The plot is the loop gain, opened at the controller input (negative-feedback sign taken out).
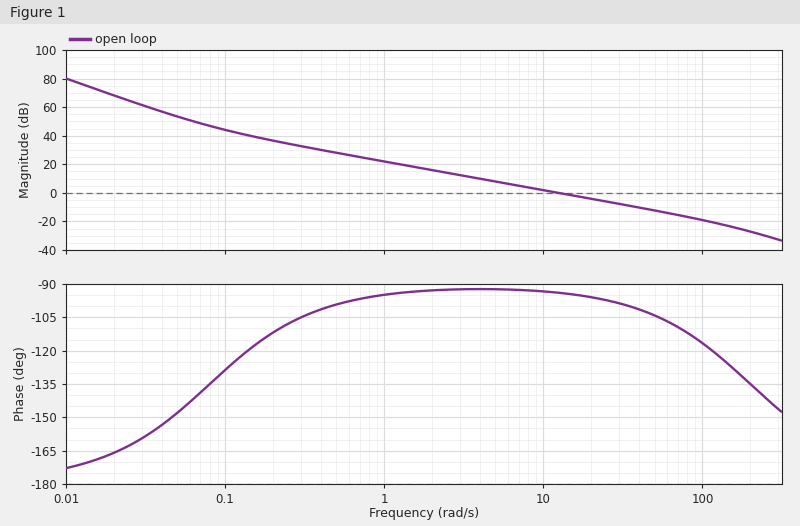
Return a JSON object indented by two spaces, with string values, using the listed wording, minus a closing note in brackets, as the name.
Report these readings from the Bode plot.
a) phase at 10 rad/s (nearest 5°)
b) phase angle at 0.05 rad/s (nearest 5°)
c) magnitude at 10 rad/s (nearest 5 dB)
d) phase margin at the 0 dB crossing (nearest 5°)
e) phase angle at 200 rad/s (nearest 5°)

{
  "phase at 10 rad/s": "-95°",
  "phase angle at 0.05 rad/s": "-150°",
  "magnitude at 10 rad/s": "0 dB",
  "phase margin at the 0 dB crossing": "85°",
  "phase angle at 200 rad/s": "-135°"
}
